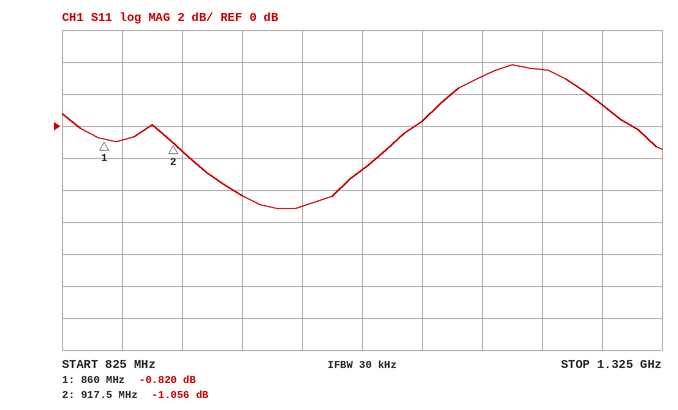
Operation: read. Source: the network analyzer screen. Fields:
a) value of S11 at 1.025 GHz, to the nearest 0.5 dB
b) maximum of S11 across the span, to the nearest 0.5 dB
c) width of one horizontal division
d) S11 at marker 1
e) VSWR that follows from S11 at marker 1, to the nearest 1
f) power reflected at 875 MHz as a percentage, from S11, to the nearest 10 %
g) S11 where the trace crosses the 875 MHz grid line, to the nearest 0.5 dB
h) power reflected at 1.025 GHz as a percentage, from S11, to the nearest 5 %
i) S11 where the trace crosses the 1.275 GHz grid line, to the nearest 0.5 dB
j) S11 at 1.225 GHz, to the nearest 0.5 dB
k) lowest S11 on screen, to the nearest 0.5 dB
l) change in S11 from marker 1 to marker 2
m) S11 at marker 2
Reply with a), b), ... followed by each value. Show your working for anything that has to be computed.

a) -5.0 dB
b) 4.0 dB
c) 50 MHz
d) -0.820 dB
e) (1 + 0.9099)/(1 − 0.9099) ≈ 21
f) 10^(-1/10) ≈ 79.4 %, so 80 % to the nearest 10 %
g) -1.0 dB
h) 10^(-5/10) ≈ 31.6 %, so 30 % to the nearest 5 %
i) 1.5 dB
j) 3.5 dB
k) -5.0 dB
l) -1.056 − (-0.82) = -0.236 dB
m) -1.056 dB
